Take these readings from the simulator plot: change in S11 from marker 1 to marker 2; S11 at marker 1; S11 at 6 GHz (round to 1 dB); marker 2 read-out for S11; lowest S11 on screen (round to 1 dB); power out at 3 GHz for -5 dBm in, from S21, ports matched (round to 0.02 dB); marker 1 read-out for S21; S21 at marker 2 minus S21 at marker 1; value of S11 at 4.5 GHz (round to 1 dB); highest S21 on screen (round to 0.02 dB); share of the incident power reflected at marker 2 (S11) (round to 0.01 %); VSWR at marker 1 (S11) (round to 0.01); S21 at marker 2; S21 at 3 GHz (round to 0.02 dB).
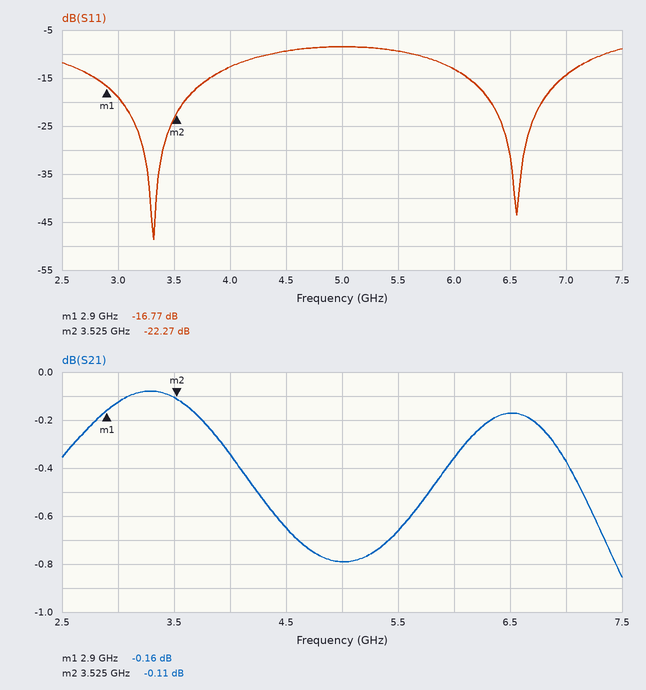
-5.50 dB
-16.77 dB
-13 dB
-22.27 dB
-49 dB
-5.12 dBm
-0.16 dB
0.05 dB
-9 dB
-0.08 dB
0.59 %
1.34
-0.11 dB
-0.12 dB
